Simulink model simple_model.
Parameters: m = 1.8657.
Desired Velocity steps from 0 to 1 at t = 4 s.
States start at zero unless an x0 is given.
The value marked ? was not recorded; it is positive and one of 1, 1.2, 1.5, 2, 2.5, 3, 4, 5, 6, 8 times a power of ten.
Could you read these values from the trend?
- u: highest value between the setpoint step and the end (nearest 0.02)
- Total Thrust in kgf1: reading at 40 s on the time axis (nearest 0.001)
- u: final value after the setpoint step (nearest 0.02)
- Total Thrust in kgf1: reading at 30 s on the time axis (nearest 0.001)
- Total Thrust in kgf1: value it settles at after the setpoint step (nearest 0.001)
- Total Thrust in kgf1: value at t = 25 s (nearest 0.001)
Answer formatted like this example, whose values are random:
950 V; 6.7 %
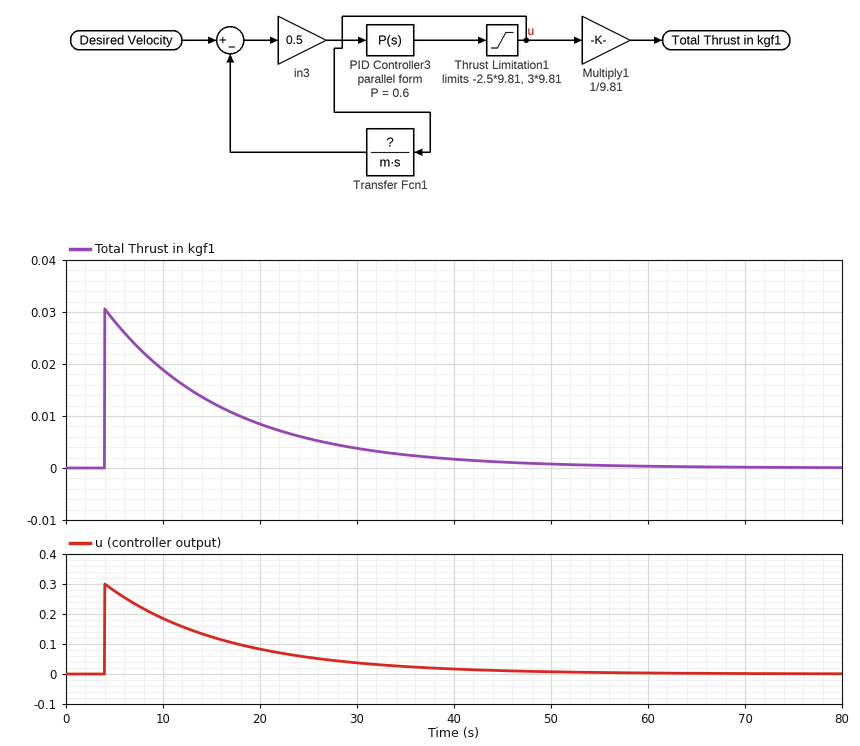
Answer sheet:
0.30; 0.002; 0.00; 0.004; 0.000; 0.006
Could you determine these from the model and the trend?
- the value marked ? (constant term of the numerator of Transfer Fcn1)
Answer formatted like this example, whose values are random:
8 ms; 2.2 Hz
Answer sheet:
0.5
